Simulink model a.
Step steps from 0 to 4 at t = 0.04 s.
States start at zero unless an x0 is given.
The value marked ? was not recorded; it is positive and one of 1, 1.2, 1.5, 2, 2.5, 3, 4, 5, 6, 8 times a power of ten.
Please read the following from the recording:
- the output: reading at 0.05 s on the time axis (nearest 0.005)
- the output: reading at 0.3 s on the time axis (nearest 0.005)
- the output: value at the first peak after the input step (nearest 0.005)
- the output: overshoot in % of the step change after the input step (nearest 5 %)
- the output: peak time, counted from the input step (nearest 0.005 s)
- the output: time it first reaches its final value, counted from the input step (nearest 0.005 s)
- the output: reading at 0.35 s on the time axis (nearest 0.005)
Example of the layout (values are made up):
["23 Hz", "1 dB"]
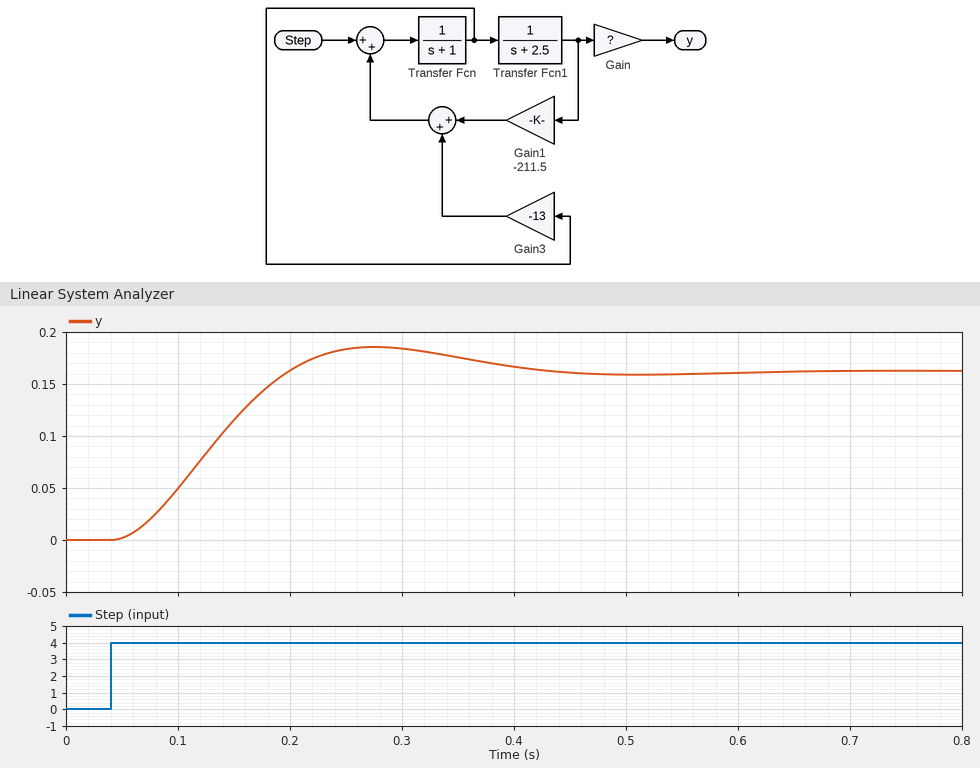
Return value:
["0.000", "0.185", "0.185", "15 %", "0.235 s", "0.160 s", "0.175"]
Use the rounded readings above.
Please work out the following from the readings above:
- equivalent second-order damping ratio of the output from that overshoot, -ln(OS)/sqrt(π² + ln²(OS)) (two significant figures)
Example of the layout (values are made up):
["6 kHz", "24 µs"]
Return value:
["0.52"]
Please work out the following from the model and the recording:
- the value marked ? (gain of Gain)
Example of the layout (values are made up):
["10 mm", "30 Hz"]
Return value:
["10"]
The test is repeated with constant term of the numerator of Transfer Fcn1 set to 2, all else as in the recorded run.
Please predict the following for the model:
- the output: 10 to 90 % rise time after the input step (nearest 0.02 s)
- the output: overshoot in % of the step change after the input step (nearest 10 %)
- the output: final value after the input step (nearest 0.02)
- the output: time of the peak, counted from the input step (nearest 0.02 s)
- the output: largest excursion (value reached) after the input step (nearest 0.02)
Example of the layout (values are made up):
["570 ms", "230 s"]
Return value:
["0.06 s", "30 %", "0.18", "0.16 s", "0.22"]
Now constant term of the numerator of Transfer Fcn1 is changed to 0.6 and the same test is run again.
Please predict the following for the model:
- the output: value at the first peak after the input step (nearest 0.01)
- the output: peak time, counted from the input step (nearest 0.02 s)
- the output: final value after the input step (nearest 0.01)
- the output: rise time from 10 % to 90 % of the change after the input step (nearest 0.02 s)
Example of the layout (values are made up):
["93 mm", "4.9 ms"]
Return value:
["0.16", "0.32 s", "0.15", "0.16 s"]
